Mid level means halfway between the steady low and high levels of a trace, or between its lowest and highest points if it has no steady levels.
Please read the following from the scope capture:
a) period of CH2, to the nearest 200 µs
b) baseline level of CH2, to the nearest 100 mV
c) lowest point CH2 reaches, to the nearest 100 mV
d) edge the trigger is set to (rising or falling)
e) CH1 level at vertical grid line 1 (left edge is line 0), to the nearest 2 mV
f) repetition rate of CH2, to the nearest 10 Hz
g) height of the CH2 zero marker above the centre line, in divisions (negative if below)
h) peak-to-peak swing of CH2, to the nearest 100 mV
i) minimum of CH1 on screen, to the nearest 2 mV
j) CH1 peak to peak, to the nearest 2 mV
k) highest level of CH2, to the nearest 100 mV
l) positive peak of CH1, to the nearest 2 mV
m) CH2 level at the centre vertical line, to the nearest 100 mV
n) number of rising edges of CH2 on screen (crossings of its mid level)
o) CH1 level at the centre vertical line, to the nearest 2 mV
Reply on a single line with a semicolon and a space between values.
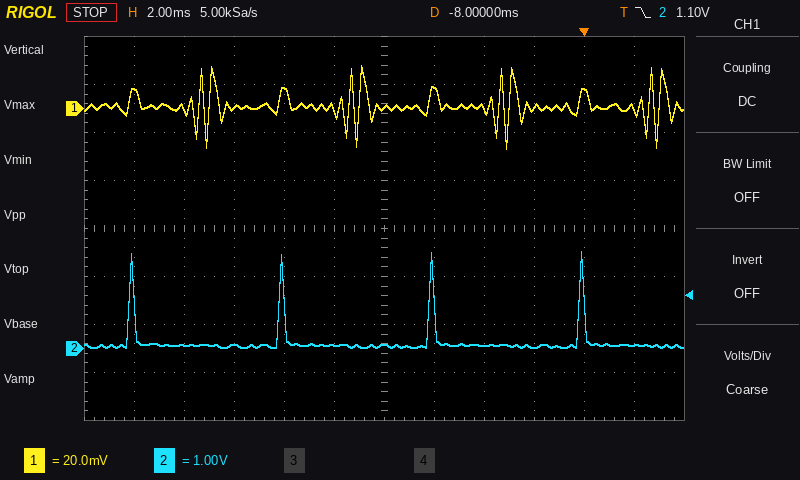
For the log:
6.0 ms; 100 mV; 0.0 V; falling; 8 mV; 170 Hz; -2.5 div; 2.0 V; -16 mV; 34 mV; 2.0 V; 18 mV; 100 mV; 4; 0 mV
